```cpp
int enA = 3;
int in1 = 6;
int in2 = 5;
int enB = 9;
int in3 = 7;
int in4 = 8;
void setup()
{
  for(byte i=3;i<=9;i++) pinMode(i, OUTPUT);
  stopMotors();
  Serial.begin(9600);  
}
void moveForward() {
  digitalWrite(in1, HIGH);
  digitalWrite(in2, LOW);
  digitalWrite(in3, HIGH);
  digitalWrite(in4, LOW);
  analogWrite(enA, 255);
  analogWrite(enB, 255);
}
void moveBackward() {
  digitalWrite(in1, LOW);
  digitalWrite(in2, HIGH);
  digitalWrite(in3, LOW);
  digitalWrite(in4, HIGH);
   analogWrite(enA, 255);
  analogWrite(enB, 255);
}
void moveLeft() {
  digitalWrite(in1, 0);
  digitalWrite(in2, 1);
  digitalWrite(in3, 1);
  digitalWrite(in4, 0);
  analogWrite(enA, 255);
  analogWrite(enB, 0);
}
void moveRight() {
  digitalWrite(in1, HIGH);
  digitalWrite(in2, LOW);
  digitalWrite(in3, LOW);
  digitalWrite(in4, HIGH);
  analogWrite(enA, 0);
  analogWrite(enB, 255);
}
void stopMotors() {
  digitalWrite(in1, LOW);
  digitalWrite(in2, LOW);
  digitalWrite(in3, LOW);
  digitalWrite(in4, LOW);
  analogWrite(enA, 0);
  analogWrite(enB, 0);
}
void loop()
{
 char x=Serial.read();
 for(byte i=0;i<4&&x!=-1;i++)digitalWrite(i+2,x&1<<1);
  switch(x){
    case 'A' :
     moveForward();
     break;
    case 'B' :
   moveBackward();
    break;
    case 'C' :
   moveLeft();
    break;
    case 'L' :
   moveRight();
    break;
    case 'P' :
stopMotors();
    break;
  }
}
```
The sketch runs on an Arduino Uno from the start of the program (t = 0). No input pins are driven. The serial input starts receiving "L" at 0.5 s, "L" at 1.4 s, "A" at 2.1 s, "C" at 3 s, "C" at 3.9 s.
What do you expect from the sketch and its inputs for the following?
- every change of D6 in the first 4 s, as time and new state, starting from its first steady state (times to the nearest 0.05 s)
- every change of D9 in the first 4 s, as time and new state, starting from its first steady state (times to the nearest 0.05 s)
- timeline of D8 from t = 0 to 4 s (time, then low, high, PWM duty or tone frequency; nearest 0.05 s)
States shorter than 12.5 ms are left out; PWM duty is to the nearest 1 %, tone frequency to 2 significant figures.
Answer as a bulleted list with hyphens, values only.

- 0 s low; 0.5 s high; 3 s low
- 0 s low; 0.5 s high; 3 s low
- 0 s low; 0.5 s high; 2.1 s low
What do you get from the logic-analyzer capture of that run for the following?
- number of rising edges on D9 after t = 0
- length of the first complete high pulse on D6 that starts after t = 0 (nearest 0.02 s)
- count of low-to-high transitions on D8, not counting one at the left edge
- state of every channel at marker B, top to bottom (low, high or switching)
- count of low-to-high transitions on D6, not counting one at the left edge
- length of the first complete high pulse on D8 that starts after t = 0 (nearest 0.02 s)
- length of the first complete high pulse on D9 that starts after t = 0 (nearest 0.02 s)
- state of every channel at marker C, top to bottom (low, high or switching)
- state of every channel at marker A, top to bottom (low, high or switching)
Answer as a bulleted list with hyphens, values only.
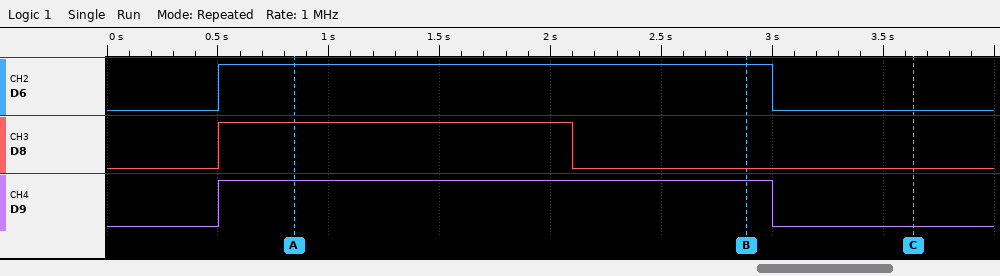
- 1
- 2.50 s
- 1
- D6 high, D8 low, D9 high
- 1
- 1.60 s
- 2.50 s
- D6 low, D8 low, D9 low
- D6 high, D8 high, D9 high
